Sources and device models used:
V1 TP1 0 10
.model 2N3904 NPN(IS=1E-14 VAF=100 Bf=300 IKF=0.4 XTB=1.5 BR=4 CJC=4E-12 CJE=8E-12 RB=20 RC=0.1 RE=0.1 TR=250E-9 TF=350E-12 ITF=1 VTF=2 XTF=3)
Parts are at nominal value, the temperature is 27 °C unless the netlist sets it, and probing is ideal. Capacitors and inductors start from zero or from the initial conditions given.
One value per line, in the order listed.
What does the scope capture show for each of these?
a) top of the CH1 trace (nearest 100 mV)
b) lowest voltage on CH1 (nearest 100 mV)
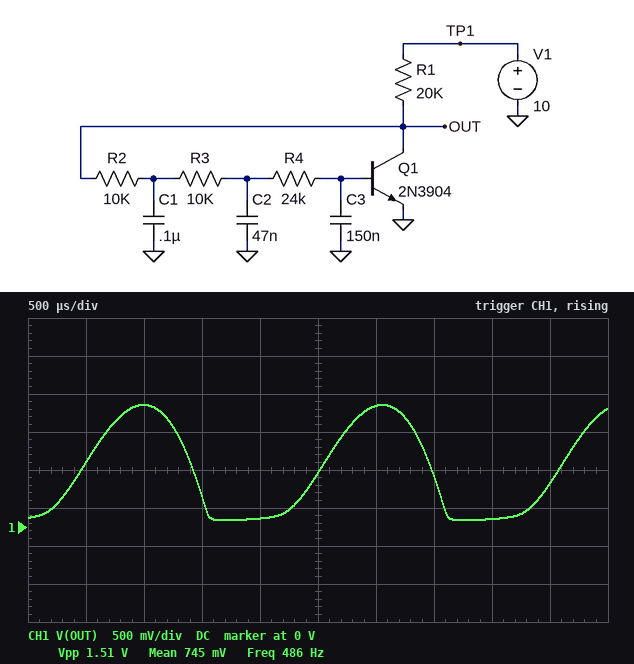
1.6 V
100 mV
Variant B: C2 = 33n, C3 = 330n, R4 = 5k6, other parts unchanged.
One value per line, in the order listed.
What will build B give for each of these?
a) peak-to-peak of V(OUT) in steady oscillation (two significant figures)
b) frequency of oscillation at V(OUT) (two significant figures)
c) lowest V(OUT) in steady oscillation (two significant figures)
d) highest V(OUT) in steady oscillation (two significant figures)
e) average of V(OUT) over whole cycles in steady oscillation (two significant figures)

1.2 V
650 Hz
100 mV
1.3 V
690 mV
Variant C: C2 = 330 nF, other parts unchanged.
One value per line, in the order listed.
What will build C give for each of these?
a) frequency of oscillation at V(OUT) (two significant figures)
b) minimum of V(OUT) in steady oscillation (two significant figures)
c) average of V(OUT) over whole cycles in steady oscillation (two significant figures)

250 Hz
100 mV
720 mV
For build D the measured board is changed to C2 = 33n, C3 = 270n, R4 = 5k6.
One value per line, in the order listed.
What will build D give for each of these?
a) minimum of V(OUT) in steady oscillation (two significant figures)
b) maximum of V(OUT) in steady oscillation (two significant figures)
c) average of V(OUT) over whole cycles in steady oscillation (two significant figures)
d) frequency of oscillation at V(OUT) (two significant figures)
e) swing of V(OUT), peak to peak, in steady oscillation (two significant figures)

95 mV
1.3 V
690 mV
710 Hz
1.2 V
